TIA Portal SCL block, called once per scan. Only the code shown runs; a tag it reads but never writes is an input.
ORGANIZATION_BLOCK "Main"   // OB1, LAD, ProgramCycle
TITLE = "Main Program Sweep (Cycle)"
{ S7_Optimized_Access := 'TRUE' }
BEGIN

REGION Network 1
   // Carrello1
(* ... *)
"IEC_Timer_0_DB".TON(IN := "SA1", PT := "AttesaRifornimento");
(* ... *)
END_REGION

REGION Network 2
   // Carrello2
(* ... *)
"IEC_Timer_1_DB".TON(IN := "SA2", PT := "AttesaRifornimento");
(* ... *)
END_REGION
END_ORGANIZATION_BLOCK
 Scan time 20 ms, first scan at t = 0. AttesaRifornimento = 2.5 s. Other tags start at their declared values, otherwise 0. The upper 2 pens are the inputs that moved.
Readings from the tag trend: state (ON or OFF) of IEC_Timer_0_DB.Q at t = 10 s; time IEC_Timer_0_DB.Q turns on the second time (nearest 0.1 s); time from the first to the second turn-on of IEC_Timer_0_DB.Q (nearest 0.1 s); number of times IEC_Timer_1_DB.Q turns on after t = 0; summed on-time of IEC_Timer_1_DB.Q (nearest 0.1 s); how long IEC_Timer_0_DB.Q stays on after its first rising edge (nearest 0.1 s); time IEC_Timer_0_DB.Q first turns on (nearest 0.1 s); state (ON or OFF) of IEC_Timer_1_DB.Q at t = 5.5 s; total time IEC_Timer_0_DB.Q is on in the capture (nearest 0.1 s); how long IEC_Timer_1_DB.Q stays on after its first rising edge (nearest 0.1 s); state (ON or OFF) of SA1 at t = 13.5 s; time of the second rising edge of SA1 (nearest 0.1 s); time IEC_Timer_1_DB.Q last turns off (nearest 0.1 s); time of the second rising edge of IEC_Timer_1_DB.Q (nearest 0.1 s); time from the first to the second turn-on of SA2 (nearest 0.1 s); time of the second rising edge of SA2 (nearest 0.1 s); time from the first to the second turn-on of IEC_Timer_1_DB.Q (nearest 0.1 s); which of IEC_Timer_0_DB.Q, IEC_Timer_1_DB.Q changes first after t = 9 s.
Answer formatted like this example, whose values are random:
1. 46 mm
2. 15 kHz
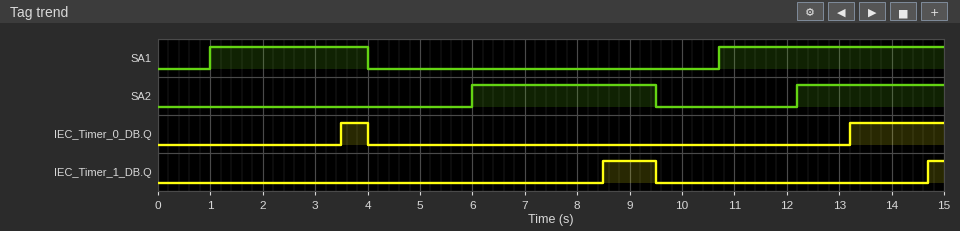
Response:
1. OFF
2. 13.2 s
3. 9.7 s
4. 2
5. 1.3 s
6. 0.5 s
7. 3.5 s
8. OFF
9. 2.3 s
10. 1.0 s
11. ON
12. 10.7 s
13. 9.5 s
14. 14.7 s
15. 6.2 s
16. 12.2 s
17. 6.2 s
18. IEC_Timer_1_DB.Q
